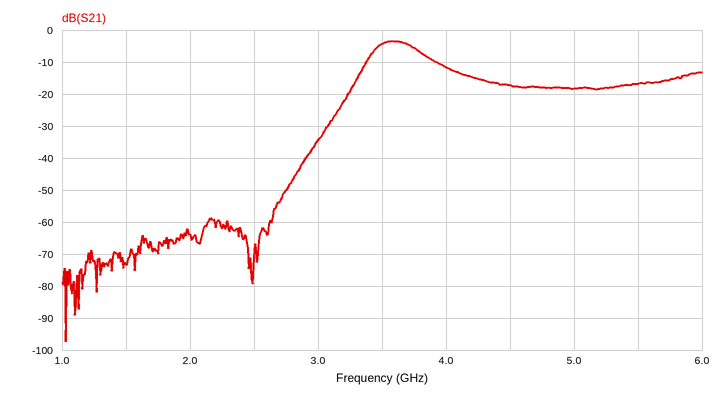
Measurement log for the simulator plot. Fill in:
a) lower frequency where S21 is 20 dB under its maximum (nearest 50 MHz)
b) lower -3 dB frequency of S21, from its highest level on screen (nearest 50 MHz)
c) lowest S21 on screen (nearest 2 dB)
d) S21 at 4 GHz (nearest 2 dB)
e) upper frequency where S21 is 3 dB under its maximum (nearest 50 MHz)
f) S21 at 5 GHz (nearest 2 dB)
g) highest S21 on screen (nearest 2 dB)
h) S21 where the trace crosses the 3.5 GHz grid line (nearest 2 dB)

3.20 GHz
3.45 GHz
-98 dB
-12 dB
3.80 GHz
-18 dB
-4 dB
-4 dB
